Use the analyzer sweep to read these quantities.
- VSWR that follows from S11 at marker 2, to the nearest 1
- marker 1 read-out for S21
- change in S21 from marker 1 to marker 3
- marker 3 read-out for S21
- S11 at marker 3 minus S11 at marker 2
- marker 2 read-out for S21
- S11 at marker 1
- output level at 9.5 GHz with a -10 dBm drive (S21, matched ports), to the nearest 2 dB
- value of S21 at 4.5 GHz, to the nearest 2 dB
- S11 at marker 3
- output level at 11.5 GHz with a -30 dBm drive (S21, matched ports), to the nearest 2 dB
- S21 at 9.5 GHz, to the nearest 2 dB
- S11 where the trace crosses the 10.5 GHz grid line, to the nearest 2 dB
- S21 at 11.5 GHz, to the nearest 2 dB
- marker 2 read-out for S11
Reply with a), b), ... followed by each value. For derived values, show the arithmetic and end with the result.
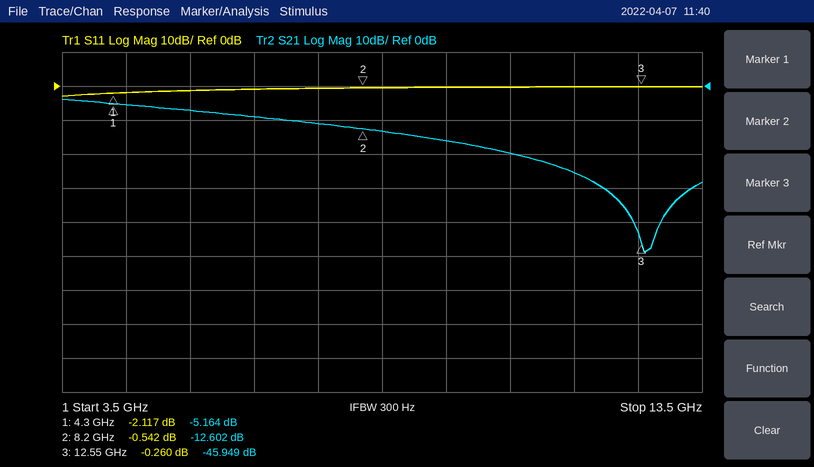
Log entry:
a) (1 + 0.9395)/(1 − 0.9395) ≈ 32
b) -5.164 dB
c) -45.949 − (-5.164) = -40.785 dB
d) -45.949 dB
e) -0.26 − (-0.542) = 0.282 dB
f) -12.602 dB
g) -2.117 dB
h) -10 dBm + (-16 dB) = -26 dBm
i) -6 dB
j) -0.260 dB
k) -30 dBm + (-26 dB) = -56 dBm
l) -16 dB
m) 0 dB
n) -26 dB
o) -0.542 dB
